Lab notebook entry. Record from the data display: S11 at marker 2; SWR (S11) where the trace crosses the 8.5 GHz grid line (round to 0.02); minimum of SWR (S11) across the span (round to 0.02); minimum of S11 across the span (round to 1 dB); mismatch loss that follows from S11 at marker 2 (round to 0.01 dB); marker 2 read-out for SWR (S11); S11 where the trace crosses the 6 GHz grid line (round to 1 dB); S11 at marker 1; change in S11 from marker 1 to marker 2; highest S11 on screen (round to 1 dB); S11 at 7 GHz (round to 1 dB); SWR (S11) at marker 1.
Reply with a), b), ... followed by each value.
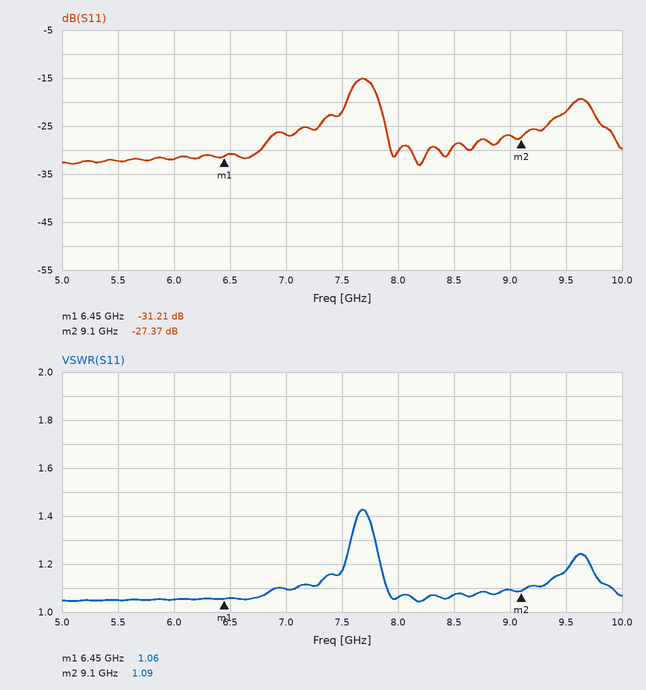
a) -27.37 dB
b) 1.08
c) 1.04
d) -33 dB
e) 0.01 dB
f) 1.09
g) -32 dB
h) -31.21 dB
i) 3.84 dB
j) -15 dB
k) -27 dB
l) 1.06
